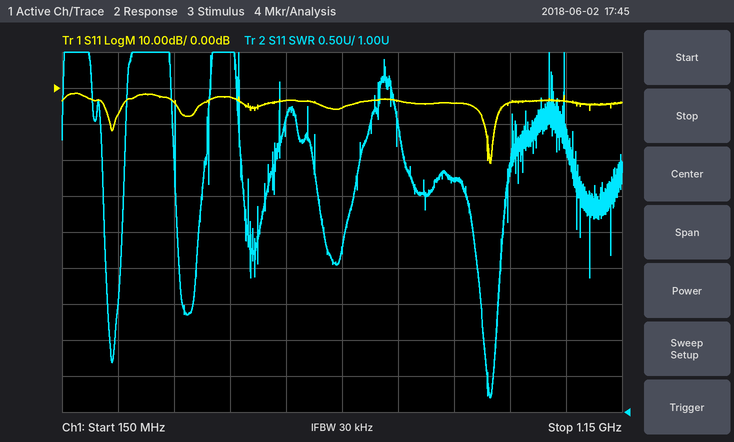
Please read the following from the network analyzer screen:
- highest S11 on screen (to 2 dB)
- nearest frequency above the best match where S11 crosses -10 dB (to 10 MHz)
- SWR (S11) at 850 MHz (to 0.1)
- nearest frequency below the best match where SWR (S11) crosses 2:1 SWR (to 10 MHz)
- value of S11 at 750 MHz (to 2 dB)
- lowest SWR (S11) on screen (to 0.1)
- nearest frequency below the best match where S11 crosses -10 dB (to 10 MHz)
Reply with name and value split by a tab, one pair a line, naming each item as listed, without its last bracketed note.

highest S11 on screen	-2 dB
nearest frequency above the best match where S11 crosses -10 dB	920 MHz
SWR (S11) at 850 MHz	4.2
nearest frequency below the best match where SWR (S11) crosses 2:1 SWR	900 MHz
value of S11 at 750 MHz	-4 dB
lowest SWR (S11) on screen	1.2
nearest frequency below the best match where S11 crosses -10 dB	900 MHz
